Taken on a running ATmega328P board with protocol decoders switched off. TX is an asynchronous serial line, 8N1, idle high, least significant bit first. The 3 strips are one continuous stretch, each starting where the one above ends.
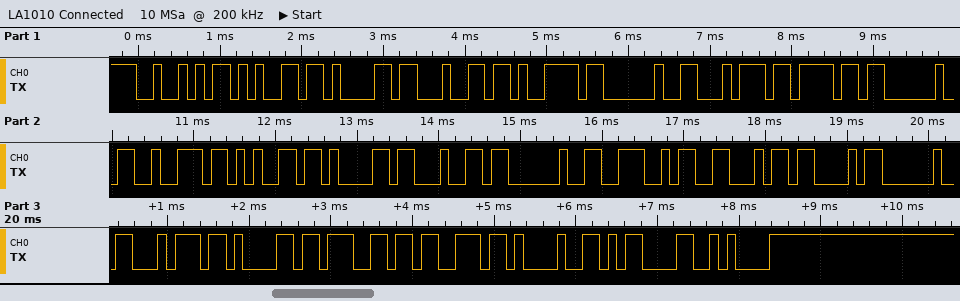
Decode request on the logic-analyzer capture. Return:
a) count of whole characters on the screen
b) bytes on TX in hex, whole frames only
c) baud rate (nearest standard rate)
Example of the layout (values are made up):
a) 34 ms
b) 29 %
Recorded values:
a) 25
b) 52 65 61 64 79 20 74 6F 20 72 65 61 64 20 4E 46 43 20 74 61 67 73 21 0D 0A
c) 9600 baud
